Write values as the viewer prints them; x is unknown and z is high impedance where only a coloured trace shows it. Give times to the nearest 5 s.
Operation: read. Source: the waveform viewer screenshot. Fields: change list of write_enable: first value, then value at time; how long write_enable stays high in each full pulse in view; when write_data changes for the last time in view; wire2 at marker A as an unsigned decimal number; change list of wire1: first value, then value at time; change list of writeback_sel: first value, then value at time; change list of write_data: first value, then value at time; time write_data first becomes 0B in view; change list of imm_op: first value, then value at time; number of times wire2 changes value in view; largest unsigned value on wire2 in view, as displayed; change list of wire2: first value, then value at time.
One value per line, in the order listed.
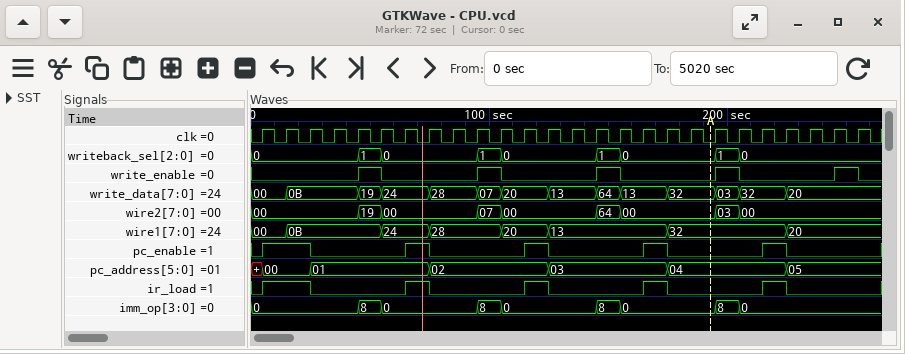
0, 1 at 45 s, 0 at 55 s, 1 at 95 s, 0 at 105 s, 1 at 145 s, 0 at 155 s, 1 at 195 s, 0 at 205 s, 1 at 245 s, 0 at 255 s
10 s, 10 s, 10 s, 10 s, 10 s
225 s
0
00, 0B at 15 s, 24 at 55 s, 28 at 75 s, 20 at 105 s, 13 at 125 s, 32 at 175 s, 20 at 225 s
0, 1 at 45 s, 0 at 55 s, 1 at 95 s, 0 at 105 s, 1 at 145 s, 0 at 155 s, 1 at 195 s, 0 at 205 s
00, 0B at 15 s, 19 at 45 s, 24 at 55 s, 28 at 75 s, 07 at 95 s, 20 at 105 s, 13 at 125 s, 64 at 145 s, 13 at 155 s, 32 at 175 s, 03 at 195 s, 32 at 205 s, 20 at 225 s
15 s
0, 8 at 45 s, 0 at 55 s, 8 at 95 s, 0 at 105 s, 8 at 145 s, 0 at 155 s, 8 at 195 s, 0 at 205 s
8
64
00, 19 at 45 s, 00 at 55 s, 07 at 95 s, 00 at 105 s, 64 at 145 s, 00 at 155 s, 03 at 195 s, 00 at 205 s
